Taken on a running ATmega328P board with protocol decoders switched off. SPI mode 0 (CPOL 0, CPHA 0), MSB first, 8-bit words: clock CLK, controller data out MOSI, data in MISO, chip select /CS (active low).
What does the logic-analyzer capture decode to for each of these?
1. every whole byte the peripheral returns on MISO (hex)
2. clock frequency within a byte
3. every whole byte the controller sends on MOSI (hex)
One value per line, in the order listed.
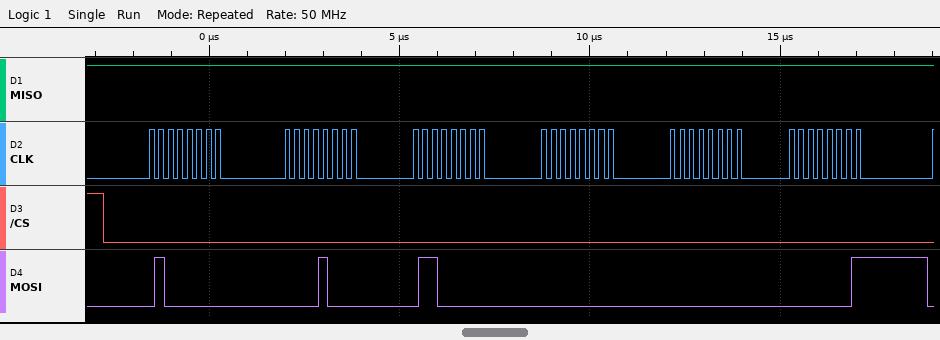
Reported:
FF FF FF FF FF FF
4 MHz
40 08 60 00 00 01
